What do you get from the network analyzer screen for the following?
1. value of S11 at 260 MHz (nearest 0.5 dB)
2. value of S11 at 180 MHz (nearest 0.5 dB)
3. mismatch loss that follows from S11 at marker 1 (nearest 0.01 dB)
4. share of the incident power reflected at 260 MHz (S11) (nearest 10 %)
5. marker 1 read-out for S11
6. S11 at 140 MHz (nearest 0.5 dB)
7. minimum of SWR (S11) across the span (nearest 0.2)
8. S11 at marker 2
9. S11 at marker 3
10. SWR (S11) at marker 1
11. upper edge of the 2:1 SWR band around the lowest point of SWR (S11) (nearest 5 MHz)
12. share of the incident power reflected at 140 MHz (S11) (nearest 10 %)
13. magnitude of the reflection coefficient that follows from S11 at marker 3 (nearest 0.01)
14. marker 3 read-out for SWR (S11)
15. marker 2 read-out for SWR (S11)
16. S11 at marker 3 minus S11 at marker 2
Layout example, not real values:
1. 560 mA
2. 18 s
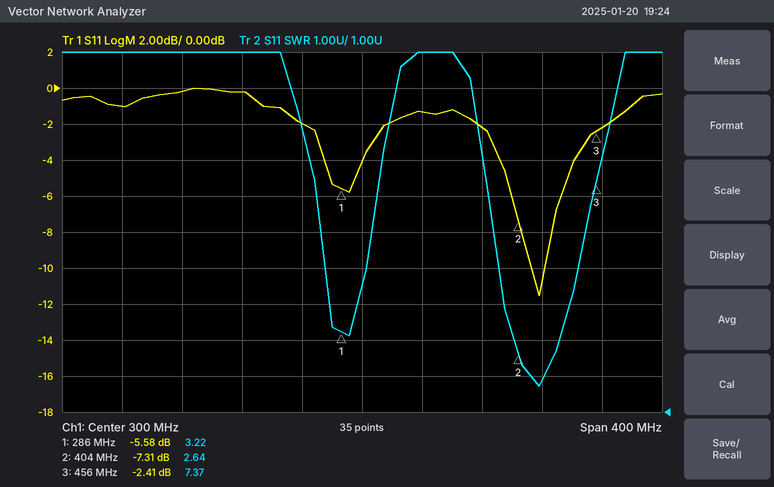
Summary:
1. -2.0 dB
2. 0.0 dB
3. 1.41 dB
4. 60 %
5. -5.58 dB
6. -1.0 dB
7. 1.8
8. -7.31 dB
9. -2.41 dB
10. 3.22
11. 420 MHz
12. 80 %
13. 0.76
14. 7.37
15. 2.64
16. 4.90 dB
